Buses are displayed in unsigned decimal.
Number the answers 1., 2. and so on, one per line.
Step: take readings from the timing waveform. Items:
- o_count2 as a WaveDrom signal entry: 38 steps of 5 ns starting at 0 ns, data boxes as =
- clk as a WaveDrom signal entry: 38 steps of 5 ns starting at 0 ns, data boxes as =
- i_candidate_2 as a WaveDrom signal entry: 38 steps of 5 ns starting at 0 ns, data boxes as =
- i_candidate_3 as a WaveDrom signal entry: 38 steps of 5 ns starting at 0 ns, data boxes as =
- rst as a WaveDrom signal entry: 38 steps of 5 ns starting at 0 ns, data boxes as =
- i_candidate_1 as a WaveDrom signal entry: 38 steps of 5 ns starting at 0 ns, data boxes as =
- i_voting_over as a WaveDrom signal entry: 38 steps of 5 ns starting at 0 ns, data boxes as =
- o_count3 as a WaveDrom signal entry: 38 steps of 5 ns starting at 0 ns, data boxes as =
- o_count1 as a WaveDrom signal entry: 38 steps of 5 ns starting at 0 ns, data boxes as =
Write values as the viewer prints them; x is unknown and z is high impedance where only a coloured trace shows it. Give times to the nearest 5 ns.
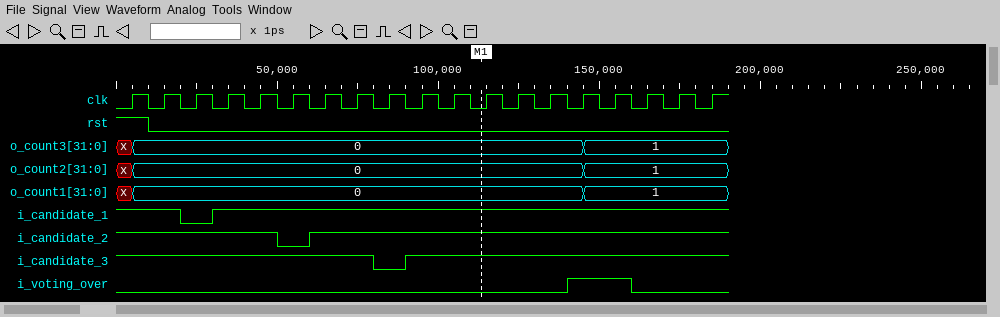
1. {name: 'o_count2', wave: 'x=...........................=........', data: '0 1'}
2. {name: 'clk', wave: '01010101010101010101010101010101010101'}
3. {name: 'i_candidate_2', wave: '1.........0.1.........................'}
4. {name: 'i_candidate_3', wave: '1...............0.1...................'}
5. {name: 'rst', wave: '1.0...................................'}
6. {name: 'i_candidate_1', wave: '1...0.1...............................'}
7. {name: 'i_voting_over', wave: '0...........................1...0.....'}
8. {name: 'o_count3', wave: 'x=...........................=........', data: '0 1'}
9. {name: 'o_count1', wave: 'x=...........................=........', data: '0 1'}
